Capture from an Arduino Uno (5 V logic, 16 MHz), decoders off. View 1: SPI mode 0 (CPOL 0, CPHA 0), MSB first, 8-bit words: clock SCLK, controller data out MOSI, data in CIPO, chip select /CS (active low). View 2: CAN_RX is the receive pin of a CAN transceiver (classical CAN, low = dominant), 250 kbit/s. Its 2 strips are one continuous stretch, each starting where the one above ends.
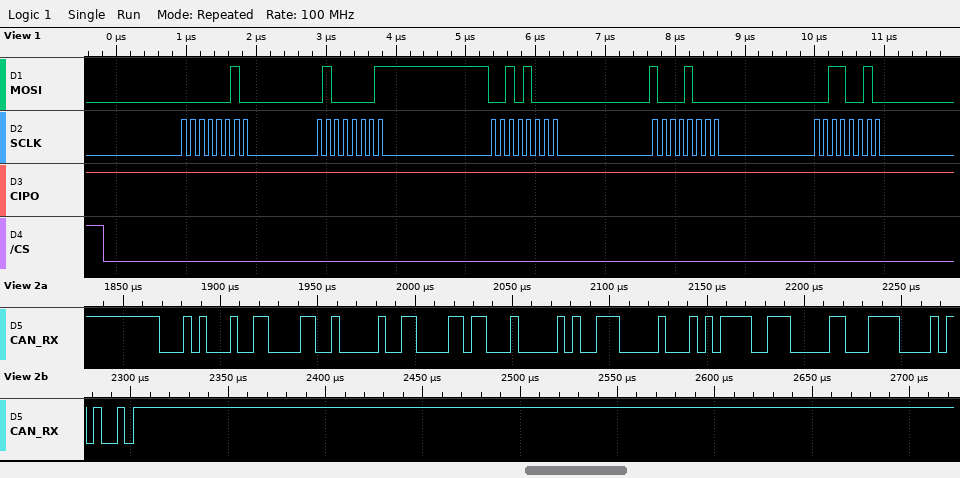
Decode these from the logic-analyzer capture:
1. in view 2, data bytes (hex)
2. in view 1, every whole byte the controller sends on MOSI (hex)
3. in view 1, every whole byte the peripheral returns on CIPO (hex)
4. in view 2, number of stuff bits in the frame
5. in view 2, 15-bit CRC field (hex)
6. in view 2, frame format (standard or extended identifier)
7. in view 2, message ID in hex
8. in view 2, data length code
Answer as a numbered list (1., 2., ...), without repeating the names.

1. C4 09 C0 2B CE 08
2. 0x02 0x41 0x28 0x88 0x32
3. 0xFF 0xFF 0xFF 0xFF 0xFF
4. 4
5. 0x7854
6. extended
7. 0x05103203
8. 6
